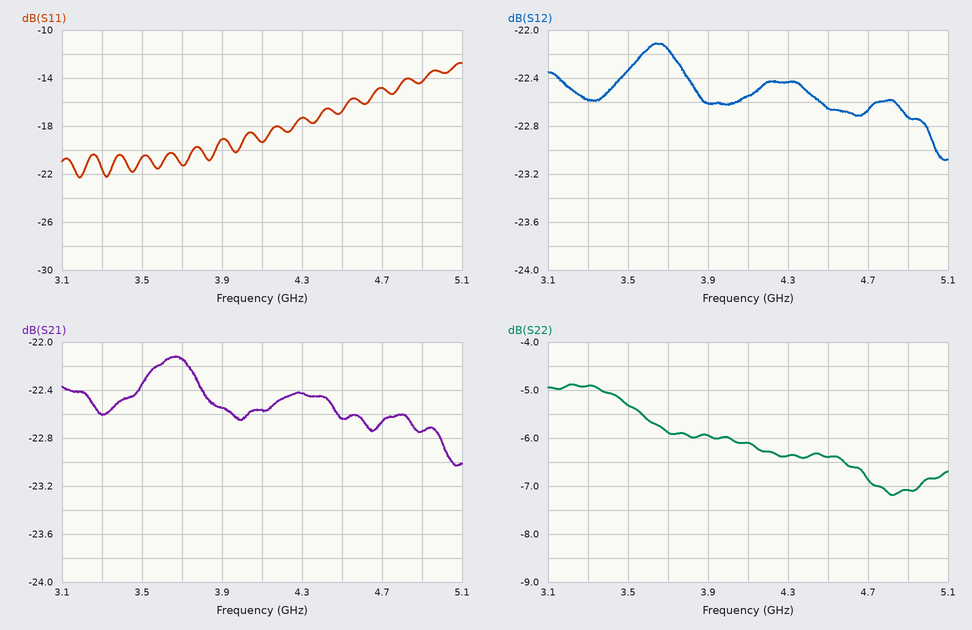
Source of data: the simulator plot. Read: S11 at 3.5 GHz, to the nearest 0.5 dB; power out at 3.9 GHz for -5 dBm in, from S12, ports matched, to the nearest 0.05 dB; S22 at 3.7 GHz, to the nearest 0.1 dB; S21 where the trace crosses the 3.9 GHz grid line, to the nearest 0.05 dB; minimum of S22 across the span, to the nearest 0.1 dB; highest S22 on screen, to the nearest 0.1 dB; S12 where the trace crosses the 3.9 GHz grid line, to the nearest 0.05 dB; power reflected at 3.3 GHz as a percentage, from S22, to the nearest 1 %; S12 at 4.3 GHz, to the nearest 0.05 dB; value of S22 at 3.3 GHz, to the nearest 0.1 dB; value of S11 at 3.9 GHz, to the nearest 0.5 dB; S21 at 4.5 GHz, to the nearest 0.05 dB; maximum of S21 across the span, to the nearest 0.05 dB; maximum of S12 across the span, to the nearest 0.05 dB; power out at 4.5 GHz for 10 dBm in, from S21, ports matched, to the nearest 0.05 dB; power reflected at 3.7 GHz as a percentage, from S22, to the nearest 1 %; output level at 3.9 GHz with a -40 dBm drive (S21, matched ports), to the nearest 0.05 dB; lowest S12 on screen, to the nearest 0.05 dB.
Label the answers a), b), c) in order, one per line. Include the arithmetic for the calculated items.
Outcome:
a) -20.5 dB
b) -5 dBm + (-22.60 dB) = -27.60 dBm
c) -5.9 dB
d) -22.55 dB
e) -7.2 dB
f) -4.9 dB
g) -22.60 dB
h) 10^(-4.9/10) ≈ 32 %
i) -22.45 dB
j) -4.9 dB
k) -19.0 dB
l) -22.65 dB
m) -22.10 dB
n) -22.10 dB
o) 10 dBm + (-22.65 dB) = -12.65 dBm
p) 10^(-5.9/10) ≈ 26 %
q) -40 dBm + (-22.55 dB) = -62.55 dBm
r) -23.10 dB
